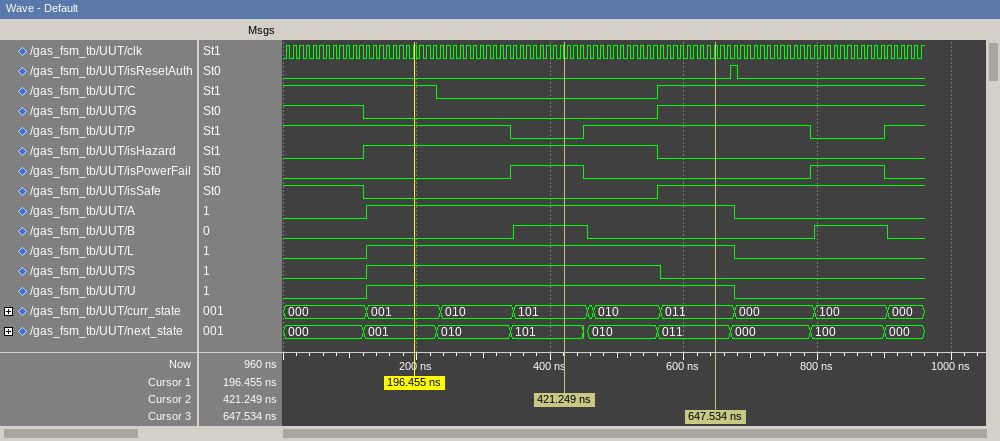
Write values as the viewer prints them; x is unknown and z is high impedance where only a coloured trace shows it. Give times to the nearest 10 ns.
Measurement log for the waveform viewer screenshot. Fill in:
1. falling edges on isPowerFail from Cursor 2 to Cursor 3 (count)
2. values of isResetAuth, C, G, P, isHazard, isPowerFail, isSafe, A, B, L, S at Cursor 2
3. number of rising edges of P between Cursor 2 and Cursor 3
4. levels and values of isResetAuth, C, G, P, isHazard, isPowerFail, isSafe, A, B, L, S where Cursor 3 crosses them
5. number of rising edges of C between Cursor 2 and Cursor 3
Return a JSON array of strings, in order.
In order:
["1", "isResetAuth=0, C=0, G=0, P=0, isHazard=1, isPowerFail=1, isSafe=0, A=1, B=1, L=1, S=1", "1", "isResetAuth=0, C=1, G=1, P=1, isHazard=0, isPowerFail=0, isSafe=1, A=1, B=0, L=1, S=0", "1"]
